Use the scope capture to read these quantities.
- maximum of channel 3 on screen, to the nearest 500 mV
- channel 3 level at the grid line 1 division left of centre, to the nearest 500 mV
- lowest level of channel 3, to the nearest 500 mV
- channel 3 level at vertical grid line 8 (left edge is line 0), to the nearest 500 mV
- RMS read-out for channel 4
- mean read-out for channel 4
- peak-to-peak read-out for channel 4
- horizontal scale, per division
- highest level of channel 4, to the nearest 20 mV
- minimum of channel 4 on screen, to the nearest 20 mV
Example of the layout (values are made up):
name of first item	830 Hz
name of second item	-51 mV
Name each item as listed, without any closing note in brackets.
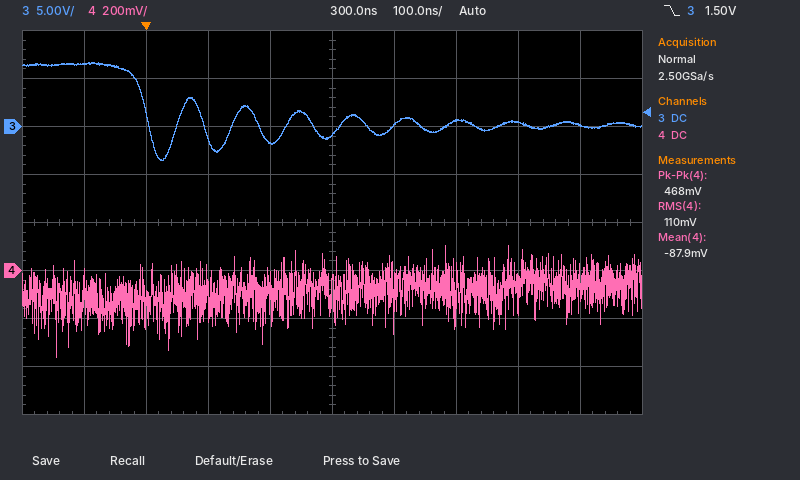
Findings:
maximum of channel 3 on screen, to the nearest 500 mV	6.5 V
channel 3 level at the grid line 1 division left of centre, to the nearest 500 mV	-1.5 V
lowest level of channel 3, to the nearest 500 mV	-3.5 V
channel 3 level at vertical grid line 8 (left edge is line 0), to the nearest 500 mV	500 mV
RMS read-out for channel 4	110 mV
mean read-out for channel 4	-87.9 mV
peak-to-peak read-out for channel 4	468 mV
horizontal scale, per division	100 ns
highest level of channel 4, to the nearest 20 mV	100 mV
minimum of channel 4 on screen, to the nearest 20 mV	-360 mV
